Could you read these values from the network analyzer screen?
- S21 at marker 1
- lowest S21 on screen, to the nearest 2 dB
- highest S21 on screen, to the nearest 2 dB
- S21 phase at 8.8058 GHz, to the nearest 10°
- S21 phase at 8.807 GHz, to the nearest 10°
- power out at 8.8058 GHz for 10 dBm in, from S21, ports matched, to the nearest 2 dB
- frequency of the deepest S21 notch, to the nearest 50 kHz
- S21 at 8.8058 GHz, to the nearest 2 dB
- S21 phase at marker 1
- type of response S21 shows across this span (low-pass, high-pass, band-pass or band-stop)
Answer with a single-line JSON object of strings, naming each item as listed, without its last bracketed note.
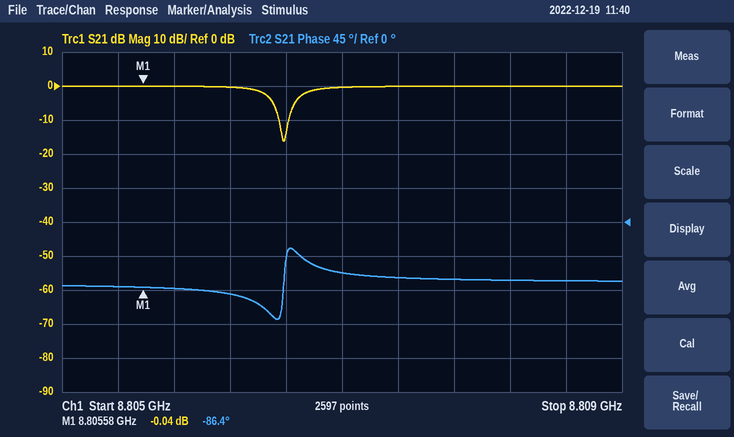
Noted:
{"S21 at marker 1": "-0.04 dB", "lowest S21 on screen, to the nearest 2 dB": "-16 dB", "highest S21 on screen, to the nearest 2 dB": "0 dB", "S21 phase at 8.8058 GHz, to the nearest 10°": "-90°", "S21 phase at 8.807 GHz, to the nearest 10°": "-70°", "power out at 8.8058 GHz for 10 dBm in, from S21, ports matched, to the nearest 2 dB": "10 dBm", "frequency of the deepest S21 notch, to the nearest 50 kHz": "8.80660 GHz", "S21 at 8.8058 GHz, to the nearest 2 dB": "0 dB", "S21 phase at marker 1": "-86.4°", "type of response S21 shows across this span": "band-stop"}
